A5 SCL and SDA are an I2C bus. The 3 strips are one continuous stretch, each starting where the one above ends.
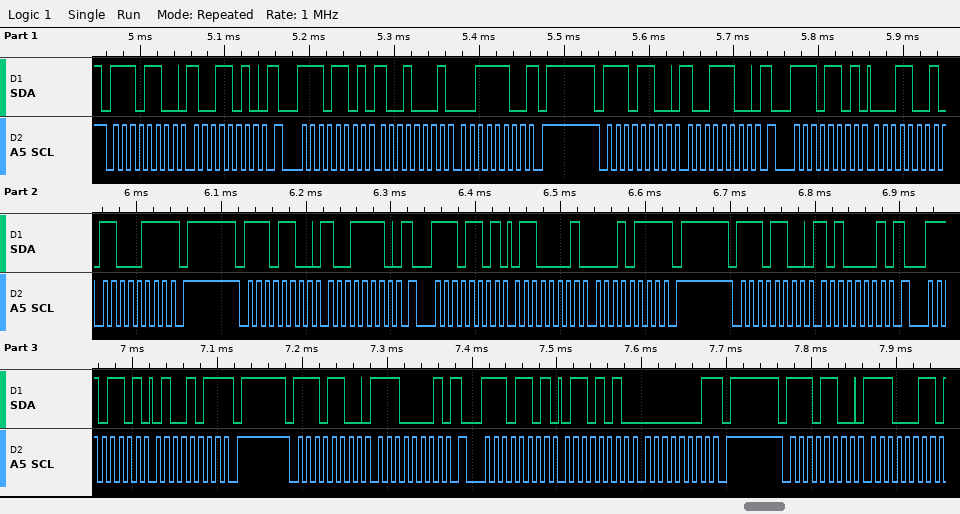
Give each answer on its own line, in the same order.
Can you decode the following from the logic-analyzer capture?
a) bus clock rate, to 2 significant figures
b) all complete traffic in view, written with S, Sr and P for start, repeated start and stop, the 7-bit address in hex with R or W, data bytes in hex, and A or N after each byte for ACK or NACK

100 kHz
S 76W A 9A A Sr 76R A 91 A 3C N P S 76W A 9C A Sr 76R A 19 A C7 N P S 76W A 9E A Sr 76R A 61 A 17 N P S 76W A A1 A Sr 76R A 4B N P S 76W A E1 A Sr 76R A 6A A 01 N P S 76W A E3 A
